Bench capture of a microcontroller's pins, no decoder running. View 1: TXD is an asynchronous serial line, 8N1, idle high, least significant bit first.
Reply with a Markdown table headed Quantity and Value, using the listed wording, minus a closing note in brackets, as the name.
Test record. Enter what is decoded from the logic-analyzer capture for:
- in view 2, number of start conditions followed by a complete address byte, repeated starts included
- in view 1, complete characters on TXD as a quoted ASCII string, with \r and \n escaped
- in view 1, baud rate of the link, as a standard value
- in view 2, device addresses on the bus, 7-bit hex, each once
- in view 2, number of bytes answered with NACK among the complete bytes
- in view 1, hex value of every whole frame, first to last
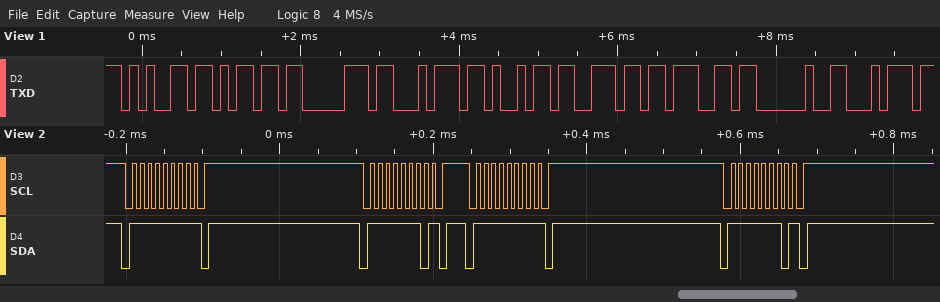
| Quantity | Value |
|---|---|
| in view 2, number of start conditions followed by a complete address byte, repeated starts included | 4 |
| in view 1, complete characters on TXD as a quoted ASCII string, with \r and \n escaped | "empting t" |
| in view 1, baud rate of the link, as a standard value | 9600 baud |
| in view 2, device addresses on the bus, 7-bit hex, each once | 0x7F |
| in view 2, number of bytes answered with NACK among the complete bytes | 4 |
| in view 1, hex value of every whole frame, first to last | 65 6D 70 74 69 6E 67 20 74 |
